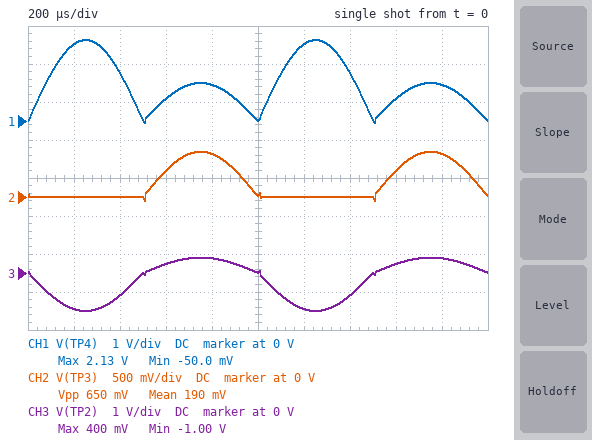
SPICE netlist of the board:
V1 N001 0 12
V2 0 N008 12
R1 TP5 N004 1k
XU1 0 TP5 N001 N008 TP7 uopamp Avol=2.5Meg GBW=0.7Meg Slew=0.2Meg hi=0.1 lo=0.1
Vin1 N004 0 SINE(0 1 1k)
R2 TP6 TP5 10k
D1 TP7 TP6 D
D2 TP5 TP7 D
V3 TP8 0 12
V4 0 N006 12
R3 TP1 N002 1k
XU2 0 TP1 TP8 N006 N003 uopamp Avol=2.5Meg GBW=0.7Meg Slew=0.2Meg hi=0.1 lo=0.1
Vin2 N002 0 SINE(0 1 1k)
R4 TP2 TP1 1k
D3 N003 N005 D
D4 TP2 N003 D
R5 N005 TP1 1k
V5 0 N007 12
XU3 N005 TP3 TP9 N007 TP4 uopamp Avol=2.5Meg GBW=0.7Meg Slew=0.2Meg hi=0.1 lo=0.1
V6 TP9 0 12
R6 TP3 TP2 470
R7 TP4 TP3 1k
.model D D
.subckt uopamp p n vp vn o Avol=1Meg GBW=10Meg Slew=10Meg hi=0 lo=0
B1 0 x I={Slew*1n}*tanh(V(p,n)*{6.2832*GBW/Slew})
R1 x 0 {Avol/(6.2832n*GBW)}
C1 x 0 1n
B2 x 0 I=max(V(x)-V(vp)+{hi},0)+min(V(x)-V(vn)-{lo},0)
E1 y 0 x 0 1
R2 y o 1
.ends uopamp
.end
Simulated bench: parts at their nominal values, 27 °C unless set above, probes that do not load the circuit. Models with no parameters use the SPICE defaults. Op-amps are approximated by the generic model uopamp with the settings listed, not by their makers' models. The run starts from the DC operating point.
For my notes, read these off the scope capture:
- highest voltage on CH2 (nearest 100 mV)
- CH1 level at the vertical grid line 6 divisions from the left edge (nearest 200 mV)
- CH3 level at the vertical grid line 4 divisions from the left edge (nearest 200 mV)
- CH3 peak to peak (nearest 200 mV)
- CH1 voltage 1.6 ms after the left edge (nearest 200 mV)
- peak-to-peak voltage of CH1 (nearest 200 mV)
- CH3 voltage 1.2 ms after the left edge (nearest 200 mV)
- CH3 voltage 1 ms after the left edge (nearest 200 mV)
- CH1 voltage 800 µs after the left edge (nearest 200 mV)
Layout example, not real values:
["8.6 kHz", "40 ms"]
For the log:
["600 mV", "2.0 V", "400 mV", "1.4 V", "600 mV", "2.2 V", "-1.0 V", "0 V", "1.0 V"]
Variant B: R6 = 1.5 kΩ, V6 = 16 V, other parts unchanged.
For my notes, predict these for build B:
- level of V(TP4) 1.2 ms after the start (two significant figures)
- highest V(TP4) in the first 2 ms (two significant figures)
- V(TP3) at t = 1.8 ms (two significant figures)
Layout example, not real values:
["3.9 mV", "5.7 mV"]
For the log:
["630 mV", "1.0 V", "680 mV"]
